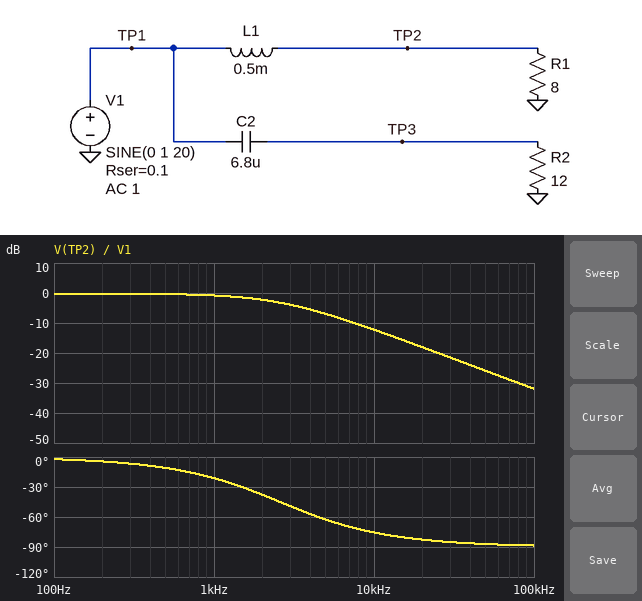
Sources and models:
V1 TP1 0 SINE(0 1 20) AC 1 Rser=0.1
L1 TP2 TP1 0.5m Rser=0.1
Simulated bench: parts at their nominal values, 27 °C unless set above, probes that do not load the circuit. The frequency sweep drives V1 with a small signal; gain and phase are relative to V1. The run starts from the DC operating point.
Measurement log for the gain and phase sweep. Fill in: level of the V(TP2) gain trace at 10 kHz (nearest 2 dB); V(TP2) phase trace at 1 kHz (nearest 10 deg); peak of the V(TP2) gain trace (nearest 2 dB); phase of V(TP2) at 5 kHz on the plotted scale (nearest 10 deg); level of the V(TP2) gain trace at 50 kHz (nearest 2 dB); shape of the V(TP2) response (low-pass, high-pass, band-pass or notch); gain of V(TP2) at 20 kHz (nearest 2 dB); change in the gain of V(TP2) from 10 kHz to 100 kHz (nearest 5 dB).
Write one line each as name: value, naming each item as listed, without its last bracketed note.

level of the V(TP2) gain trace at 10 kHz: -12 dB
V(TP2) phase trace at 1 kHz: -20 deg
peak of the V(TP2) gain trace: 0 dB
phase of V(TP2) at 5 kHz on the plotted scale: -60 deg
level of the V(TP2) gain trace at 50 kHz: -26 dB
shape of the V(TP2) response: low-pass
gain of V(TP2) at 20 kHz: -18 dB
change in the gain of V(TP2) from 10 kHz to 100 kHz: -20 dB
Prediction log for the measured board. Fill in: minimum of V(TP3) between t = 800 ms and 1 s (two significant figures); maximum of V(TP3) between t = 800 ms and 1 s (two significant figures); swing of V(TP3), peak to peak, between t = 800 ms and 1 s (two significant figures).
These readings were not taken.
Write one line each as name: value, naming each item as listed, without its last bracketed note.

minimum of V(TP3) between t = 800 ms and 1 s: -10 mV
maximum of V(TP3) between t = 800 ms and 1 s: 10 mV
swing of V(TP3), peak to peak, between t = 800 ms and 1 s: 20 mV
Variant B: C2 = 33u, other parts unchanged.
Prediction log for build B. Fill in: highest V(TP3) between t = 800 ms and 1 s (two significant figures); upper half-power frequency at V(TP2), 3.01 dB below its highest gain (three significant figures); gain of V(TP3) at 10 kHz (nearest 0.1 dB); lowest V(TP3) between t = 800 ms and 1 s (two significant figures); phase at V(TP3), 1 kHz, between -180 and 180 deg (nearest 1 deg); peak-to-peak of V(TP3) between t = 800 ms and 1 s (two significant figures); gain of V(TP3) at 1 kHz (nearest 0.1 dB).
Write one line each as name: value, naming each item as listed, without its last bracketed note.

highest V(TP3) between t = 800 ms and 1 s: 49 mV
upper half-power frequency at V(TP2), 3.01 dB below its highest gain: 2.57 kHz
gain of V(TP3) at 10 kHz: -0.1 dB
lowest V(TP3) between t = 800 ms and 1 s: -49 mV
phase at V(TP3), 1 kHz, between -180 and 180 deg: 22 deg
peak-to-peak of V(TP3) between t = 800 ms and 1 s: 98 mV
gain of V(TP3) at 1 kHz: -0.8 dB
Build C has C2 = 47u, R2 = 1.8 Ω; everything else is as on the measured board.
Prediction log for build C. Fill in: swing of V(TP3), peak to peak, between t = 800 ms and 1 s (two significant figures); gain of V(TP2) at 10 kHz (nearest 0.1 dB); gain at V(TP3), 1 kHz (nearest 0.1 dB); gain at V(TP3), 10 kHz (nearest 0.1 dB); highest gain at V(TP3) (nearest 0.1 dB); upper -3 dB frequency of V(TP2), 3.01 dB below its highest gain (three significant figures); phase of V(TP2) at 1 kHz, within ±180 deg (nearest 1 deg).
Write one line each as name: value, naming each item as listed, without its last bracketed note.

swing of V(TP3), peak to peak, between t = 800 ms and 1 s: 21 mV
gain of V(TP2) at 10 kHz: -12.6 dB
gain at V(TP3), 1 kHz: -6.8 dB
gain at V(TP3), 10 kHz: -0.6 dB
highest gain at V(TP3): -0.5 dB
upper -3 dB frequency of V(TP2), 3.01 dB below its highest gain: 2.43 kHz
phase of V(TP2) at 1 kHz, within ±180 deg: -22 deg
